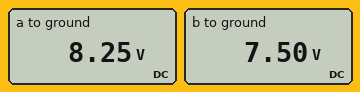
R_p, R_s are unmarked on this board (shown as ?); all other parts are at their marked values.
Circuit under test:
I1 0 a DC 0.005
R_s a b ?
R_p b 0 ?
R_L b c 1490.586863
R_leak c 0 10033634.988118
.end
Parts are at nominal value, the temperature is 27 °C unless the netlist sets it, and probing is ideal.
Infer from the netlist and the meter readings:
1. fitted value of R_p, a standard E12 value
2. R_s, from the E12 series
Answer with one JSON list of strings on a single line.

["1.5 kΩ", "150 Ω"]
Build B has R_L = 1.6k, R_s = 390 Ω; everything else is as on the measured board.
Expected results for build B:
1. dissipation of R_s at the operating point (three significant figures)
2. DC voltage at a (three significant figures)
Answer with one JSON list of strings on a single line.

["9.75 mW", "9.45 V"]
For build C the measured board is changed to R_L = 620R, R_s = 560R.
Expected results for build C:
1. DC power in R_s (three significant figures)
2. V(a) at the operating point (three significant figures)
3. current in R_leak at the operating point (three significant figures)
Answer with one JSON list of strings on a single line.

["14.0 mW", "10.3 V", "747 nA"]
